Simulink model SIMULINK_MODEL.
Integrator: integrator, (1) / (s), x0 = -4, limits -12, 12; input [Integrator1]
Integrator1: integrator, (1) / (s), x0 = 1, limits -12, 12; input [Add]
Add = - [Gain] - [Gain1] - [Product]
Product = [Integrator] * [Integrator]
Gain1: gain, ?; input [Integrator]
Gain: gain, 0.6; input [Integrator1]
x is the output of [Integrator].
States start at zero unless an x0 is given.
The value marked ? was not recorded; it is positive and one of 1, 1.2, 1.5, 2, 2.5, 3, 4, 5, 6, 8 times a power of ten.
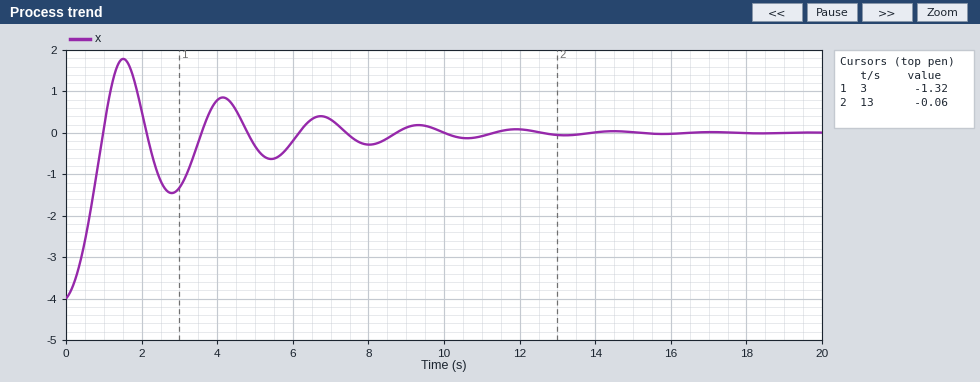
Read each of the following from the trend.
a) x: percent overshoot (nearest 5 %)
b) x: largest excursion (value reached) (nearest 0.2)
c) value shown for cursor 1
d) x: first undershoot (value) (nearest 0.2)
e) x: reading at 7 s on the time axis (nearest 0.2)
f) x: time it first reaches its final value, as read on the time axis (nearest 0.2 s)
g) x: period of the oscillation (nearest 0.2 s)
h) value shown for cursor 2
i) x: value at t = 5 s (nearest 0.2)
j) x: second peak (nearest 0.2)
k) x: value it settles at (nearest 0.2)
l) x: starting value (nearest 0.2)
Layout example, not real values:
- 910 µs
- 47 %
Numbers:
- 45 %
- 1.8
- -1.32
- -1.4
- 0.4
- 1.0 s
- 2.6 s
- -0.06
- -0.4
- 0.8
- 0.0
- -4.0
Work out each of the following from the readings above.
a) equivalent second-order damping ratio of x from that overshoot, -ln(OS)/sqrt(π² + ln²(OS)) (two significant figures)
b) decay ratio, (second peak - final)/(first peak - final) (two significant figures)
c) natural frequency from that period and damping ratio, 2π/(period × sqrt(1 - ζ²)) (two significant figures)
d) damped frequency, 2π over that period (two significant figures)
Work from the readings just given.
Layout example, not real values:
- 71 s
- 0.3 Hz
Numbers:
- 0.25
- 0.44
- 2.5 rad/s
- 2.4 rad/s
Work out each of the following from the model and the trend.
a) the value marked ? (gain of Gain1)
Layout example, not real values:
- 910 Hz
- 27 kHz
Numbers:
- 6
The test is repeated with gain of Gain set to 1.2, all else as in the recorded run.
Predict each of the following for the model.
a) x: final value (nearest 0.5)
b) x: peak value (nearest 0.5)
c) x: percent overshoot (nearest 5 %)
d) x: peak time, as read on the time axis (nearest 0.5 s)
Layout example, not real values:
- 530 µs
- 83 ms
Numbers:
- 0.0
- 1.0
- 30 %
- 1.5 s
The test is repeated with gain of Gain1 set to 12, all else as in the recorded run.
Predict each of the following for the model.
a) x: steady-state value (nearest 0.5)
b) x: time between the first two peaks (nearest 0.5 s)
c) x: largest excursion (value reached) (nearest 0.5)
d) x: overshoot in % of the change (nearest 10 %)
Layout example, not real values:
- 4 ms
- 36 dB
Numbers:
- 0.0
- 2.0 s
- 2.5
- 60 %
